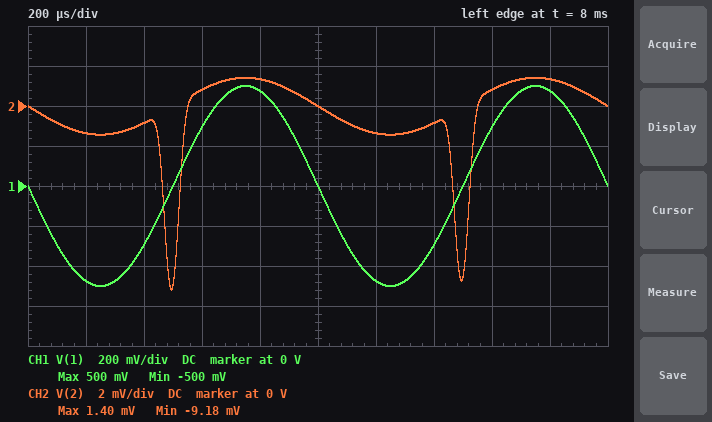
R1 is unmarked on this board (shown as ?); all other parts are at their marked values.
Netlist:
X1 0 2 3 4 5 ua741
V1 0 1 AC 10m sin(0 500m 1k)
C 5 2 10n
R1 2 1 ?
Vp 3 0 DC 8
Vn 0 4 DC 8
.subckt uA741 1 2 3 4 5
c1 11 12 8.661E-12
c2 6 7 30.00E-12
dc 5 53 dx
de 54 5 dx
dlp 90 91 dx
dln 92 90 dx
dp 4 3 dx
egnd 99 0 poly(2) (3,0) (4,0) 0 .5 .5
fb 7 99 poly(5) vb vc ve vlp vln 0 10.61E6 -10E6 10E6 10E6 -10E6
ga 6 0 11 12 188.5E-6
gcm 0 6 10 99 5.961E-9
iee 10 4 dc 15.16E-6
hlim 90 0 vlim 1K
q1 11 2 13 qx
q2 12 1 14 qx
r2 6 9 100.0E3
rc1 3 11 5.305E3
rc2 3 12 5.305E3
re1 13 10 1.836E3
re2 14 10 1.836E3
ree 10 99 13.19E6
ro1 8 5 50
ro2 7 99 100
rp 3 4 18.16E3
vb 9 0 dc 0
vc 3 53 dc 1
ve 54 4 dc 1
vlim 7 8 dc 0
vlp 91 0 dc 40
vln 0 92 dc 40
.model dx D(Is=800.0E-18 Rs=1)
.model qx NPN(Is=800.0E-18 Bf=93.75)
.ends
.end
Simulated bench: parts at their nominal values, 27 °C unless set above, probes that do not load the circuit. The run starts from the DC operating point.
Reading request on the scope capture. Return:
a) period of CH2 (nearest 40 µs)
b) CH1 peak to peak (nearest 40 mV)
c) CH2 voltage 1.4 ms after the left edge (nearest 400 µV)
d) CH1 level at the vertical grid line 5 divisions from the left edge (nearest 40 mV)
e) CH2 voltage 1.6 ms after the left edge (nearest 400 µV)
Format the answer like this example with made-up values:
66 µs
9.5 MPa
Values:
1.00 ms
1.00 V
-800 µV
0 V
800 µV
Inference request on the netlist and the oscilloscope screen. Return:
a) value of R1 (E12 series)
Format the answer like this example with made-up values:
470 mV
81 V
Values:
5.6 kΩ
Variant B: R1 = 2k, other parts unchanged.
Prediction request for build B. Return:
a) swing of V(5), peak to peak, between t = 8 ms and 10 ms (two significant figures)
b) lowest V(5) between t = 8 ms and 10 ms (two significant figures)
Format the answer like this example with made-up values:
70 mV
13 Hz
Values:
7.9 V
-350 mV
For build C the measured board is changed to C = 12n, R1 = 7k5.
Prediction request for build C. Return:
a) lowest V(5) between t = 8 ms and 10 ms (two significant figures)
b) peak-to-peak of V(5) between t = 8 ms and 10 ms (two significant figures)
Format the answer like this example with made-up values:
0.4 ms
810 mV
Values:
5.8 V
1.8 V
